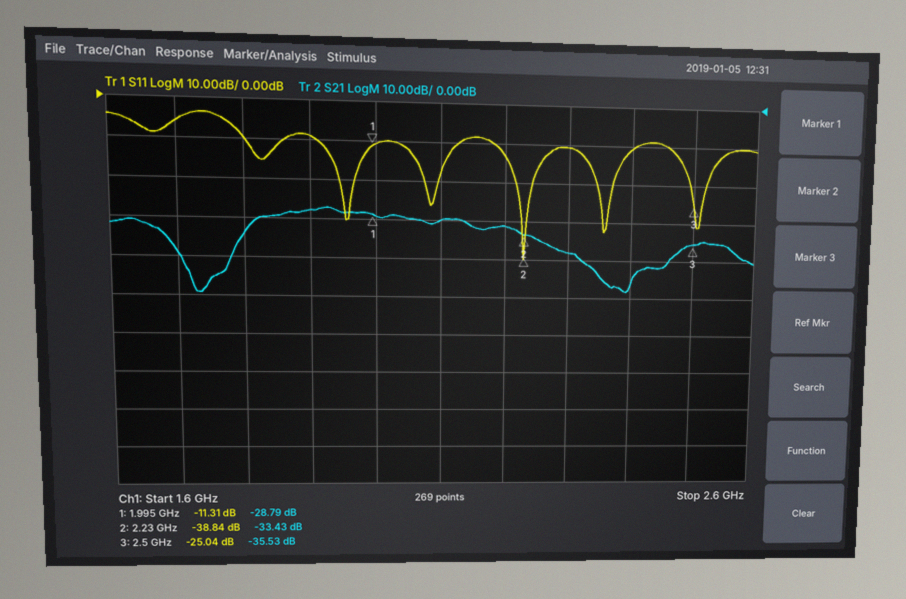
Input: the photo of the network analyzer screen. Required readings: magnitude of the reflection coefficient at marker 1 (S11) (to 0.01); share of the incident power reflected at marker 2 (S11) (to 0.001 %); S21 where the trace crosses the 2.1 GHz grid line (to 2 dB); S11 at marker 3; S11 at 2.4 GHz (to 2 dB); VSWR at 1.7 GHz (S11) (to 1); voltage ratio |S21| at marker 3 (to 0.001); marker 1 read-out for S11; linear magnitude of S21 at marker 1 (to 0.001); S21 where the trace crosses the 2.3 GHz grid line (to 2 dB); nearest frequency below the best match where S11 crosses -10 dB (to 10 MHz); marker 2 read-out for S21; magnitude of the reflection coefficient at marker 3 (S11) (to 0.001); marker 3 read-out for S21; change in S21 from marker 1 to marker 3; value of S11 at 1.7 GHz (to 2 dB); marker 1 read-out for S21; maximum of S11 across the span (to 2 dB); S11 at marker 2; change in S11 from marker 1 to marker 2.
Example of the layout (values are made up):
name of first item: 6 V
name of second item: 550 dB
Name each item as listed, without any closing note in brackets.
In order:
magnitude of the reflection coefficient at marker 1 (S11): 0.27
share of the incident power reflected at marker 2 (S11): 0.013 %
S21 where the trace crosses the 2.1 GHz grid line: -30 dB
S11 at marker 3: -25.04 dB
S11 at 2.4 GHz: -10 dB
VSWR at 1.7 GHz (S11): 3
voltage ratio |S21| at marker 3: 0.017
marker 1 read-out for S11: -11.31 dB
linear magnitude of S21 at marker 1: 0.036
S21 where the trace crosses the 2.3 GHz grid line: -38 dB
nearest frequency below the best match where S11 crosses -10 dB: 2.18 GHz
marker 2 read-out for S21: -33.43 dB
magnitude of the reflection coefficient at marker 3 (S11): 0.056
marker 3 read-out for S21: -35.53 dB
change in S21 from marker 1 to marker 3: -6.74 dB
value of S11 at 1.7 GHz: -6 dB
marker 1 read-out for S21: -28.79 dB
maximum of S11 across the span: -4 dB
S11 at marker 2: -38.84 dB
change in S11 from marker 1 to marker 2: -27.53 dB
